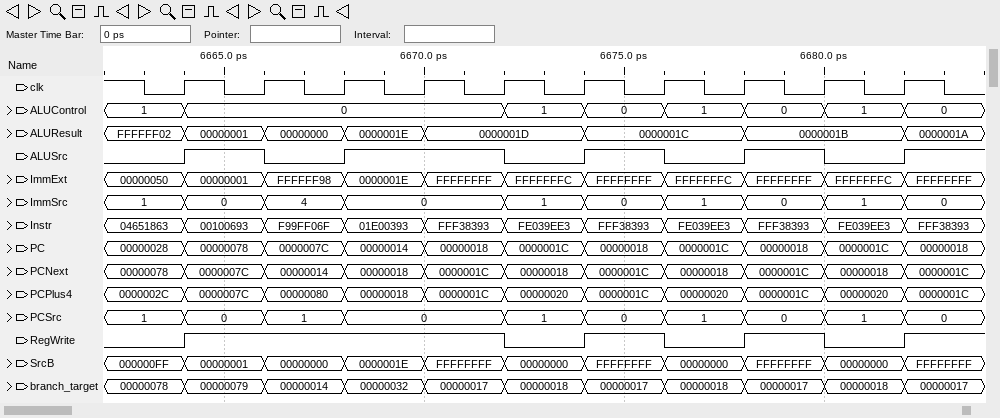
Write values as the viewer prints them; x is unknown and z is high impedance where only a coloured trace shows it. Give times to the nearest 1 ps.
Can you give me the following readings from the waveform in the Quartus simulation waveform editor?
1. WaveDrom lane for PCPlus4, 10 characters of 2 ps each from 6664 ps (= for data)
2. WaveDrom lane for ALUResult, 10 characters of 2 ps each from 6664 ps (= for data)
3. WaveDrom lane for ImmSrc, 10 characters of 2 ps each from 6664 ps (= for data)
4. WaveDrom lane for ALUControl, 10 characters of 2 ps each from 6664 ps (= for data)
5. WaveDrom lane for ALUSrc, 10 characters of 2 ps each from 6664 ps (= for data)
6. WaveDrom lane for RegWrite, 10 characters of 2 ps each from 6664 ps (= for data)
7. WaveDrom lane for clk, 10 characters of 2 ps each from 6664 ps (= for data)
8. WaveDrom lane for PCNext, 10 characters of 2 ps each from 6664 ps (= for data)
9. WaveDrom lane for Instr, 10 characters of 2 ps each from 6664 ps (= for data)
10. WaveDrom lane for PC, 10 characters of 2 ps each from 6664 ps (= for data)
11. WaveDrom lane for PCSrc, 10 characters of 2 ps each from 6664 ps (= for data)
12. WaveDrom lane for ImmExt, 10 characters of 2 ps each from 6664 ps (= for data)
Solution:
{name: 'PCPlus4', wave: '==========', data: '0000007C 00000080 00000018 0000001C 00000020 0000001C 00000020 0000001C 00000020 0000001C'}
{name: 'ALUResult', wave: '====.=.=.=', data: '00000001 00000000 0000001E 0000001D 0000001C 0000001B 0000001A'}
{name: 'ImmSrc', wave: '===.======', data: '0 4 0 1 0 1 0 1 0'}
{name: 'ALUControl', wave: '=...======', data: '0 1 0 1 0 1 0'}
{name: 'ALUSrc', wave: '101.010101'}
{name: 'RegWrite', wave: '1...010101'}
{name: 'clk', wave: 'p.........'}
{name: 'PCNext', wave: '==========', data: '0000007C 00000014 00000018 0000001C 00000018 0000001C 00000018 0000001C 00000018 0000001C'}
{name: 'Instr', wave: '==========', data: '00100693 F99FF06F 01E00393 FFF38393 FE039EE3 FFF38393 FE039EE3 FFF38393 FE039EE3 FFF38393'}
{name: 'PC', wave: '==========', data: '00000078 0000007C 00000014 00000018 0000001C 00000018 0000001C 00000018 0000001C 00000018'}
{name: 'PCSrc', wave: '===.======', data: '0 1 0 1 0 1 0 1 0'}
{name: 'ImmExt', wave: '==========', data: '00000001 FFFFFF98 0000001E FFFFFFFF FFFFFFFC FFFFFFFF FFFFFFFC FFFFFFFF FFFFFFFC FFFFFFFF'}
